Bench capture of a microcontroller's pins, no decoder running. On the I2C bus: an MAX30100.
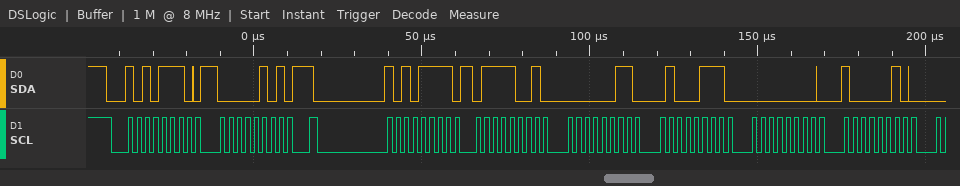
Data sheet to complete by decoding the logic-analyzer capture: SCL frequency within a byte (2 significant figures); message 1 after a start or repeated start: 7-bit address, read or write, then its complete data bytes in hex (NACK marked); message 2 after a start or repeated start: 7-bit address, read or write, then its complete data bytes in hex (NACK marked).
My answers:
400 kHz
0x57 write: 05
0x57 read: 79 03 47 00 82
